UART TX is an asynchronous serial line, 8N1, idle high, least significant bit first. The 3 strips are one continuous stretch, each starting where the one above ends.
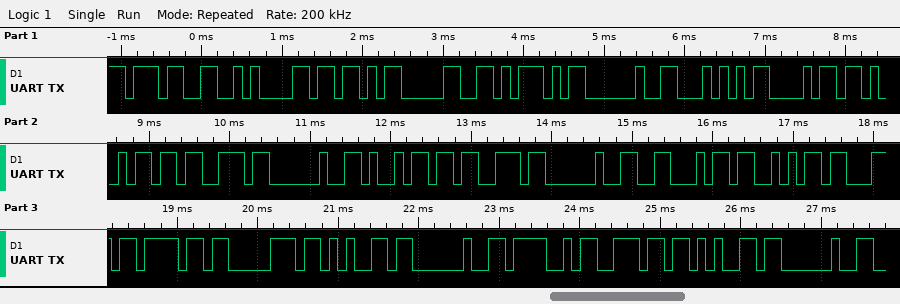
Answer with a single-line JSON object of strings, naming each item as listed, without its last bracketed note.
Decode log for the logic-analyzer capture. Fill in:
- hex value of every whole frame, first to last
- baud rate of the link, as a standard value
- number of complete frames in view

{"hex value of every whole frame, first to last": "0x37 0x0A 0x5B 0x30 0x5D 0x20 0x54 0x68 0x69 0x73 0x20 0x69 0x73 0x20 0x46 0x53 0x63 0x6F 0x70 0x65 0x20 0x4F 0x6E 0x65 0x20", "baud rate of the link, as a standard value": "9600 baud", "number of complete frames in view": "25"}
